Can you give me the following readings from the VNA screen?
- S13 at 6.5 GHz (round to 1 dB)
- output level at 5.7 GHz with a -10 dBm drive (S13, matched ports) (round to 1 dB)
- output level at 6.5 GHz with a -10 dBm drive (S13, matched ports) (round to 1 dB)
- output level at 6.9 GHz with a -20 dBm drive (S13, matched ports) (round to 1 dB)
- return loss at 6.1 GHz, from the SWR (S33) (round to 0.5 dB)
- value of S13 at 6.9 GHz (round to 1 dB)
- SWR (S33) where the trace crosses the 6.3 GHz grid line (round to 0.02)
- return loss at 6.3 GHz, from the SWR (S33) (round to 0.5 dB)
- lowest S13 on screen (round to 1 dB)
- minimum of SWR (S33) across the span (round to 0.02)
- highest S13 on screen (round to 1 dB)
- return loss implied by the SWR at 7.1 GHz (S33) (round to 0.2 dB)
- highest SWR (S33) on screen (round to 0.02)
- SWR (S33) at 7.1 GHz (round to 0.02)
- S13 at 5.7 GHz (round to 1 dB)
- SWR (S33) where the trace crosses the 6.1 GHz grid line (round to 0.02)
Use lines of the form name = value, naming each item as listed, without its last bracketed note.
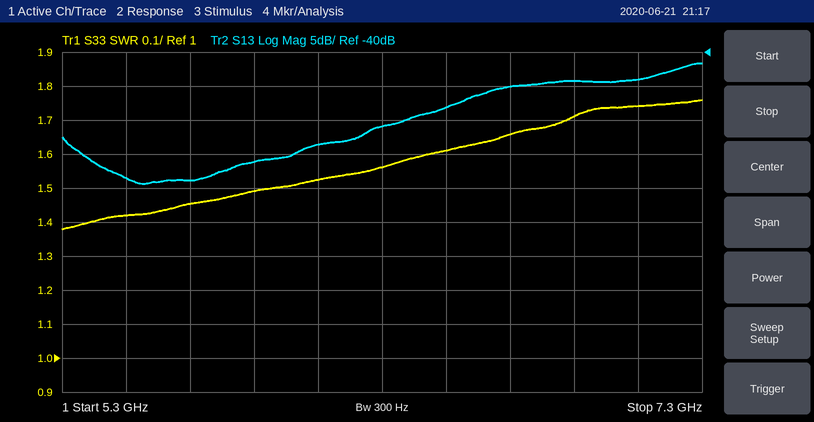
S13 at 6.5 GHz = -48 dB
output level at 5.7 GHz with a -10 dBm drive (S13, matched ports) = -69 dBm
output level at 6.5 GHz with a -10 dBm drive (S13, matched ports) = -58 dBm
output level at 6.9 GHz with a -20 dBm drive (S13, matched ports) = -64 dBm
return loss at 6.1 GHz, from the SWR (S33) = 13.5 dB
value of S13 at 6.9 GHz = -44 dB
SWR (S33) where the trace crosses the 6.3 GHz grid line = 1.56
return loss at 6.3 GHz, from the SWR (S33) = 13.0 dB
lowest S13 on screen = -59 dB
minimum of SWR (S33) across the span = 1.38
highest S13 on screen = -42 dB
return loss implied by the SWR at 7.1 GHz (S33) = 11.4 dB
highest SWR (S33) on screen = 1.76
SWR (S33) at 7.1 GHz = 1.74
S13 at 5.7 GHz = -59 dB
SWR (S33) where the trace crosses the 6.1 GHz grid line = 1.52
